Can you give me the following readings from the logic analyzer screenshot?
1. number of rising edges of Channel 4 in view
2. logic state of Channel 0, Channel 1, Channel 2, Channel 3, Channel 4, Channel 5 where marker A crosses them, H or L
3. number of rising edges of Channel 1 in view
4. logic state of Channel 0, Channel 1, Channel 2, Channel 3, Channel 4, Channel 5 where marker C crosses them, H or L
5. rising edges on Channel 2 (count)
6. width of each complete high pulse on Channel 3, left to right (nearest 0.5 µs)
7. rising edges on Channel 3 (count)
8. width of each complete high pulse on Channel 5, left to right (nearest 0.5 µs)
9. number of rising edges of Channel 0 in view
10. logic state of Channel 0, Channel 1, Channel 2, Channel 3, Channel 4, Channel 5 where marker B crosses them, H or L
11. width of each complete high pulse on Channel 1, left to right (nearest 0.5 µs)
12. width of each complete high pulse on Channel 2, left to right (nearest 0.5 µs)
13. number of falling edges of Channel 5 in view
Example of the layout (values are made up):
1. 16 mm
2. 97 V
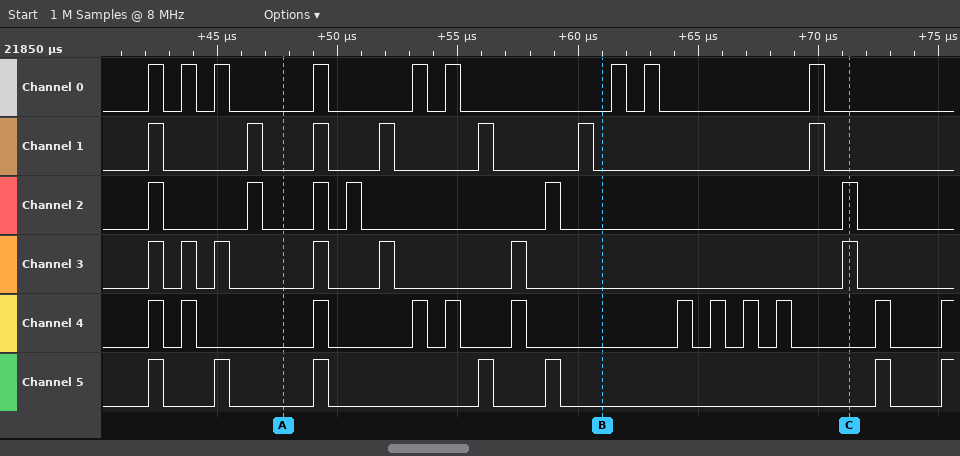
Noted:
1. 12
2. Channel 0=L, Channel 1=L, Channel 2=L, Channel 3=L, Channel 4=L, Channel 5=L
3. 7
4. Channel 0=L, Channel 1=L, Channel 2=H, Channel 3=H, Channel 4=L, Channel 5=L
5. 6
6. 0.5 µs, 0.5 µs, 0.5 µs, 0.5 µs, 0.5 µs, 0.5 µs, 0.5 µs
7. 7
8. 0.5 µs, 0.5 µs, 0.5 µs, 0.5 µs, 0.5 µs, 0.5 µs
9. 9
10. Channel 0=L, Channel 1=L, Channel 2=L, Channel 3=L, Channel 4=L, Channel 5=L
11. 0.5 µs, 0.5 µs, 0.5 µs, 0.5 µs, 0.5 µs, 0.5 µs, 0.5 µs
12. 0.5 µs, 0.5 µs, 0.5 µs, 0.5 µs, 0.5 µs, 0.5 µs
13. 6
